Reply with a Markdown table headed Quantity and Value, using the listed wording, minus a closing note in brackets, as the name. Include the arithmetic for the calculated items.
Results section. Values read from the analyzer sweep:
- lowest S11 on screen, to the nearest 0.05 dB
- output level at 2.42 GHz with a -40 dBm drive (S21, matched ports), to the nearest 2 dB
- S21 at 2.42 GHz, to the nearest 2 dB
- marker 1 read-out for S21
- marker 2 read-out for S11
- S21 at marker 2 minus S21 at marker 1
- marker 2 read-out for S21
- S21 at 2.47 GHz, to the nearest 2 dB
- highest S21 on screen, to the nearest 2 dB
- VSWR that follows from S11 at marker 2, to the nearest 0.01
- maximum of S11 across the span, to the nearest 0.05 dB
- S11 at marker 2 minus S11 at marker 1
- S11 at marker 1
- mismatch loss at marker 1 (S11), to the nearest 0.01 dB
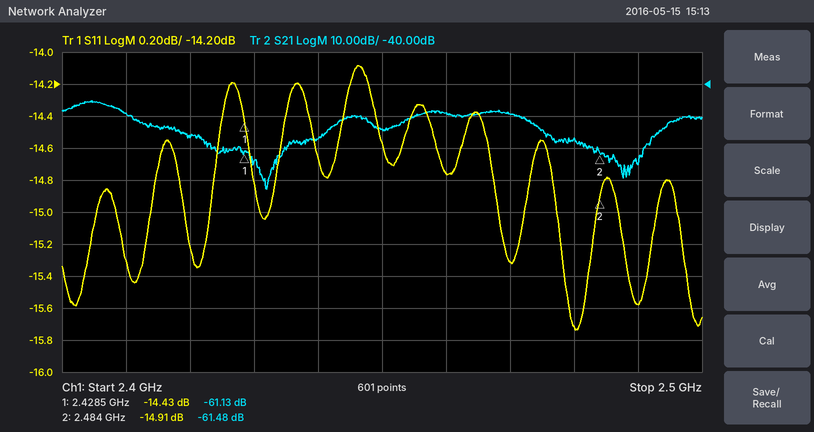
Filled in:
| Quantity | Value |
|---|---|
| lowest S11 on screen, to the nearest 0.05 dB | -15.75 dB |
| output level at 2.42 GHz with a -40 dBm drive (S21, matched ports), to the nearest 2 dB | -40 dBm + (-56 dB) = -96 dBm |
| S21 at 2.42 GHz, to the nearest 2 dB | -56 dB |
| marker 1 read-out for S21 | -61.13 dB |
| marker 2 read-out for S11 | -14.91 dB |
| S21 at marker 2 minus S21 at marker 1 | -61.48 − (-61.13) = -0.35 dB |
| marker 2 read-out for S21 | -61.48 dB |
| S21 at 2.47 GHz, to the nearest 2 dB | -50 dB |
| highest S21 on screen, to the nearest 2 dB | -46 dB |
| VSWR that follows from S11 at marker 2, to the nearest 0.01 | (1 + 0.1797)/(1 − 0.1797) ≈ 1.44 |
| maximum of S11 across the span, to the nearest 0.05 dB | -14.10 dB |
| S11 at marker 2 minus S11 at marker 1 | -14.91 − (-14.43) = -0.48 dB |
| S11 at marker 1 | -14.43 dB |
| mismatch loss at marker 1 (S11), to the nearest 0.01 dB | −10 log10(1 − 10^(-14.43/10)) ≈ 0.16 dB |
